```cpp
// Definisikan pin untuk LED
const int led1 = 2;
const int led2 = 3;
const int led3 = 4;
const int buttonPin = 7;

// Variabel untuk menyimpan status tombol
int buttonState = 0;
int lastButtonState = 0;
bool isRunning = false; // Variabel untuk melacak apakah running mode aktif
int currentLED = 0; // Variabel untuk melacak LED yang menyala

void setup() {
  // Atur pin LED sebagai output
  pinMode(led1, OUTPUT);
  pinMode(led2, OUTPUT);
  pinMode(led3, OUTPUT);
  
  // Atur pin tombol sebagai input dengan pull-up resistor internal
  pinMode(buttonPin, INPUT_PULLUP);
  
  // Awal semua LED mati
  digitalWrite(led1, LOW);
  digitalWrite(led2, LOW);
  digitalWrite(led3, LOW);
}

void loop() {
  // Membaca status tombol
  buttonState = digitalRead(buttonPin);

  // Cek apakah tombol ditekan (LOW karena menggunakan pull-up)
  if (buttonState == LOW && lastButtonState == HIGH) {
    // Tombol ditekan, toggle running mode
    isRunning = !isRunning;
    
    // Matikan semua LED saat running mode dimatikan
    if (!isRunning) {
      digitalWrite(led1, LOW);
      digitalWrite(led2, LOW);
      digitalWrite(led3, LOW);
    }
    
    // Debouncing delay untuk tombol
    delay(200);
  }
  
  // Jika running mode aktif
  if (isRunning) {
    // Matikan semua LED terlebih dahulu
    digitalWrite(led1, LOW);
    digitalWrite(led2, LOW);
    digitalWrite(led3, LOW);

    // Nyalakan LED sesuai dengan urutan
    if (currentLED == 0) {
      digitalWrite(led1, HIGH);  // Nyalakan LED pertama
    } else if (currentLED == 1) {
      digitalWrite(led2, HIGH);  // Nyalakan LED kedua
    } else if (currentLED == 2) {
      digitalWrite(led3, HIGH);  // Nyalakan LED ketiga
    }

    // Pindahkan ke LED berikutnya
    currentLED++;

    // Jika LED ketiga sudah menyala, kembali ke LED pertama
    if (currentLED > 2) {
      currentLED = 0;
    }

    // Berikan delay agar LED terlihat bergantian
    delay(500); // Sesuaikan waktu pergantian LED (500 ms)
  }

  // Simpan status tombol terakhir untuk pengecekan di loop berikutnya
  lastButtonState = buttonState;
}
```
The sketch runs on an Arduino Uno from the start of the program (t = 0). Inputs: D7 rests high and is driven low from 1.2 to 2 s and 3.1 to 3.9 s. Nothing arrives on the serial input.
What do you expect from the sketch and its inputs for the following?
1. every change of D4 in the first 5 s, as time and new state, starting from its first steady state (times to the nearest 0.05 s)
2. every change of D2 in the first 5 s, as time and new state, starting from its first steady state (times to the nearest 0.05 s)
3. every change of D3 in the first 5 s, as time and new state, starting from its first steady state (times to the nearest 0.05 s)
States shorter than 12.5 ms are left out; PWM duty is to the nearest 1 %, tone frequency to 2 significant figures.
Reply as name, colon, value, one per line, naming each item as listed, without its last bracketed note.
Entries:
every change of D4 in the first 5 s, as time and new state, starting from its first steady state: 0 s low; 2.4 s high; 2.9 s low
every change of D2 in the first 5 s, as time and new state, starting from its first steady state: 0 s low; 1.4 s high; 1.9 s low; 2.9 s high; 3.4 s low
every change of D3 in the first 5 s, as time and new state, starting from its first steady state: 0 s low; 1.9 s high; 2.4 s low
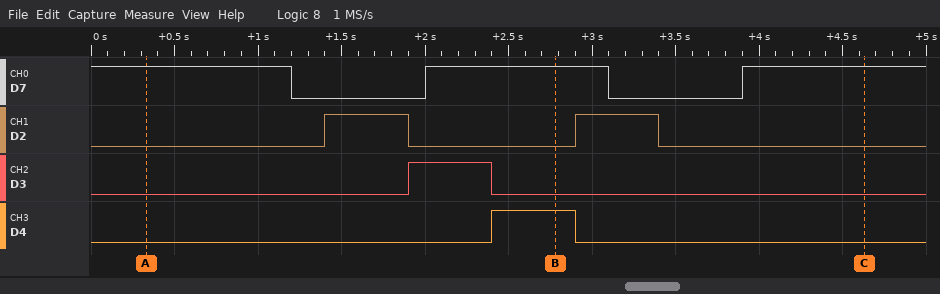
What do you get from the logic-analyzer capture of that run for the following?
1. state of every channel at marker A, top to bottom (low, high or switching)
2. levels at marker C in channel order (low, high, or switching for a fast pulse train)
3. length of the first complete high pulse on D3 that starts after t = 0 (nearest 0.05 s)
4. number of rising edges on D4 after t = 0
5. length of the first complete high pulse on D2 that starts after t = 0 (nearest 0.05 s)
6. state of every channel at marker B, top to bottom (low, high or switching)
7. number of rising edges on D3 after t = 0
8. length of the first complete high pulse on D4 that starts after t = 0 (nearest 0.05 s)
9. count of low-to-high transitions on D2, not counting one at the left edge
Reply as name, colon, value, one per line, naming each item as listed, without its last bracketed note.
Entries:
state of every channel at marker A, top to bottom: D7 high, D2 low, D3 low, D4 low
levels at marker C in channel order: D7 high, D2 low, D3 low, D4 low
length of the first complete high pulse on D3 that starts after t = 0: 0.50 s
number of rising edges on D4 after t = 0: 1
length of the first complete high pulse on D2 that starts after t = 0: 0.50 s
state of every channel at marker B, top to bottom: D7 high, D2 low, D3 low, D4 high
number of rising edges on D3 after t = 0: 1
length of the first complete high pulse on D4 that starts after t = 0: 0.50 s
count of low-to-high transitions on D2, not counting one at the left edge: 2
